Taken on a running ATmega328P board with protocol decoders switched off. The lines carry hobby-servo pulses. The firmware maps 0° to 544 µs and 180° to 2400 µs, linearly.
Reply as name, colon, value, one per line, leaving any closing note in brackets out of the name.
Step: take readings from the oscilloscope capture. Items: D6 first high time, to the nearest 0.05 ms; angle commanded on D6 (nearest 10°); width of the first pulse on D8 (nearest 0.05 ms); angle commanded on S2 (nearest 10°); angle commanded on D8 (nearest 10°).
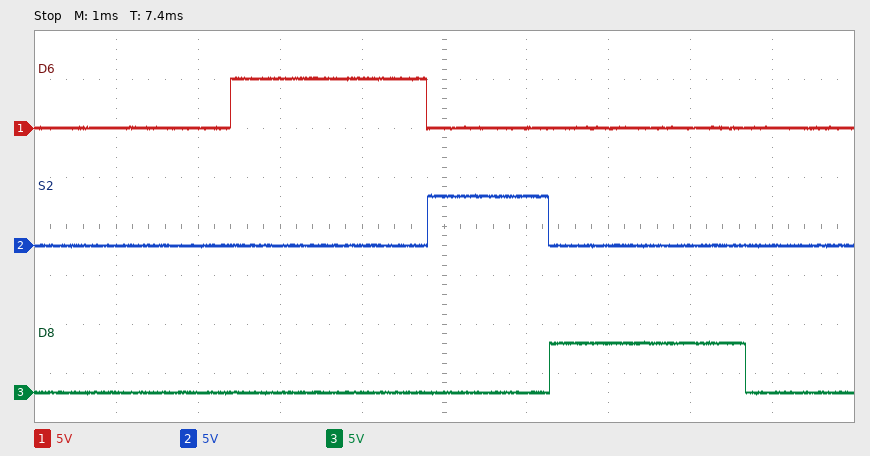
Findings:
D6 first high time, to the nearest 0.05 ms: 2.40 ms
angle commanded on D6: 180°
width of the first pulse on D8: 2.40 ms
angle commanded on S2: 90°
angle commanded on D8: 180°
